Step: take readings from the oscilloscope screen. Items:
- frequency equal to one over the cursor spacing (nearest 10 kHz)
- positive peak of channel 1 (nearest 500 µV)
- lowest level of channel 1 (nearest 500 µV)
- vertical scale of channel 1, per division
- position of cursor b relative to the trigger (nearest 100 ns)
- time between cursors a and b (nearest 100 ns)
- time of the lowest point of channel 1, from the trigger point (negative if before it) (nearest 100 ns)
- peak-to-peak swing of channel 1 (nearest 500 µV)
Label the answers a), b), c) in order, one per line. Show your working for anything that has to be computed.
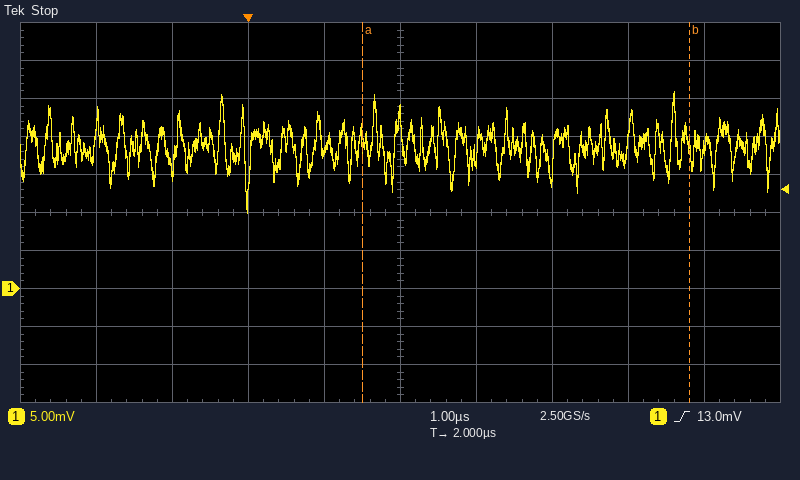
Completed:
a) 1 / 4.3 µs ≈ 230 kHz
b) 26.0 mV
c) 10.0 mV
d) 5 mV
e) +5.8 µs
f) 4.3 µs
g) 0.0 µs
h) 26.0 mV − (10.0 mV) = 16.0 mV
